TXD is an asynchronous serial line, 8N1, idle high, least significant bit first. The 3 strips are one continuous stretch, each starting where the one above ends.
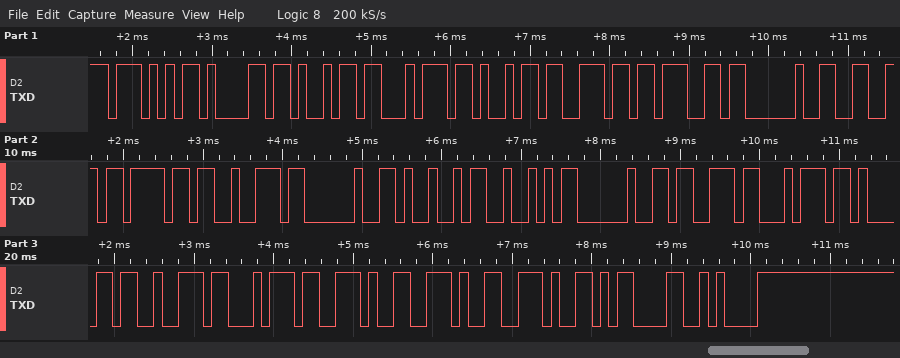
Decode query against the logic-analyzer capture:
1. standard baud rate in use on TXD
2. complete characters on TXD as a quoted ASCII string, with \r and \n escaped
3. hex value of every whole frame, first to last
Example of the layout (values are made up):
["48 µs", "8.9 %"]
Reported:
["9600 baud", "\"Waiting for IR start...\\r\\n\"", "57 61 69 74 69 6E 67 20 66 6F 72 20 49 52 20 73 74 61 72 74 2E 2E 2E 0D 0A"]
